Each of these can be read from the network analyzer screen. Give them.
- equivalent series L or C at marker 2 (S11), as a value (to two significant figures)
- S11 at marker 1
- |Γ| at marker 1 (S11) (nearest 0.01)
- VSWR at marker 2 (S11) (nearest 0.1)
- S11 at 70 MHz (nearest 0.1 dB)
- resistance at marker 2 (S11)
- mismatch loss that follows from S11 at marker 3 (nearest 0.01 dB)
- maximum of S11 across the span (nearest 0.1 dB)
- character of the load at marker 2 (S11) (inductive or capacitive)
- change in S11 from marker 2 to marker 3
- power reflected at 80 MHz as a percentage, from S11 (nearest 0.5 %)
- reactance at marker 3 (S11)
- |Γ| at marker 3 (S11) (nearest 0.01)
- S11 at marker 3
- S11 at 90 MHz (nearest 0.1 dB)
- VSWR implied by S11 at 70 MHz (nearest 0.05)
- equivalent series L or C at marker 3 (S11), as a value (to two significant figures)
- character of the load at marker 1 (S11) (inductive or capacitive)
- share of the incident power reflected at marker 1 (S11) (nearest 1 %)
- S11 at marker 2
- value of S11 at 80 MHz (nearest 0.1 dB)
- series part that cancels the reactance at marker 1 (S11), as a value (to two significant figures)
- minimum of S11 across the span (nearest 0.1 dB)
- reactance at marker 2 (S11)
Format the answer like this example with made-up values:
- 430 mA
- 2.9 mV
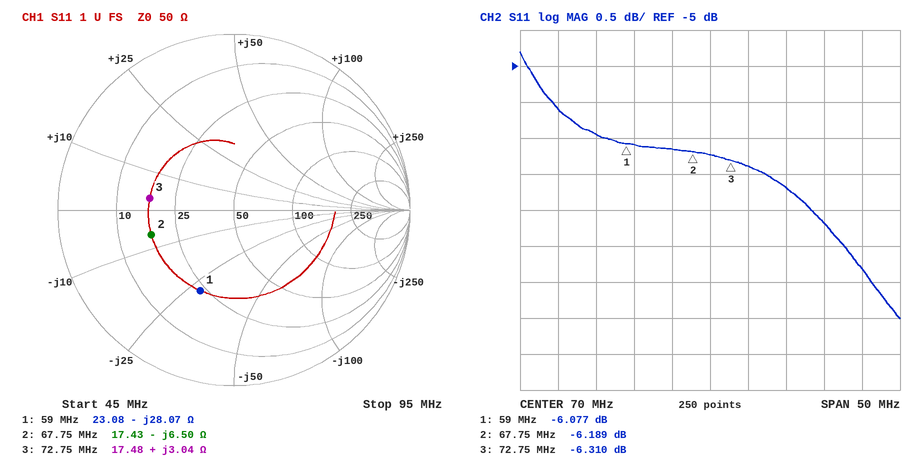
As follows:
- 360 pF
- -6.077 dB
- 0.50
- 2.9
- -6.2 dB
- 17.43 Ω
- 1.16 dB
- -4.8 dB
- capacitive
- -0.121 dB
- 21.5 %
- +3.04 Ω
- 0.48
- -6.310 dB
- -7.8 dB
- 2.90
- 6.7 nH
- capacitive
- 25 %
- -6.189 dB
- -6.7 dB
- 76 nH
- -8.5 dB
- -6.50 Ω
